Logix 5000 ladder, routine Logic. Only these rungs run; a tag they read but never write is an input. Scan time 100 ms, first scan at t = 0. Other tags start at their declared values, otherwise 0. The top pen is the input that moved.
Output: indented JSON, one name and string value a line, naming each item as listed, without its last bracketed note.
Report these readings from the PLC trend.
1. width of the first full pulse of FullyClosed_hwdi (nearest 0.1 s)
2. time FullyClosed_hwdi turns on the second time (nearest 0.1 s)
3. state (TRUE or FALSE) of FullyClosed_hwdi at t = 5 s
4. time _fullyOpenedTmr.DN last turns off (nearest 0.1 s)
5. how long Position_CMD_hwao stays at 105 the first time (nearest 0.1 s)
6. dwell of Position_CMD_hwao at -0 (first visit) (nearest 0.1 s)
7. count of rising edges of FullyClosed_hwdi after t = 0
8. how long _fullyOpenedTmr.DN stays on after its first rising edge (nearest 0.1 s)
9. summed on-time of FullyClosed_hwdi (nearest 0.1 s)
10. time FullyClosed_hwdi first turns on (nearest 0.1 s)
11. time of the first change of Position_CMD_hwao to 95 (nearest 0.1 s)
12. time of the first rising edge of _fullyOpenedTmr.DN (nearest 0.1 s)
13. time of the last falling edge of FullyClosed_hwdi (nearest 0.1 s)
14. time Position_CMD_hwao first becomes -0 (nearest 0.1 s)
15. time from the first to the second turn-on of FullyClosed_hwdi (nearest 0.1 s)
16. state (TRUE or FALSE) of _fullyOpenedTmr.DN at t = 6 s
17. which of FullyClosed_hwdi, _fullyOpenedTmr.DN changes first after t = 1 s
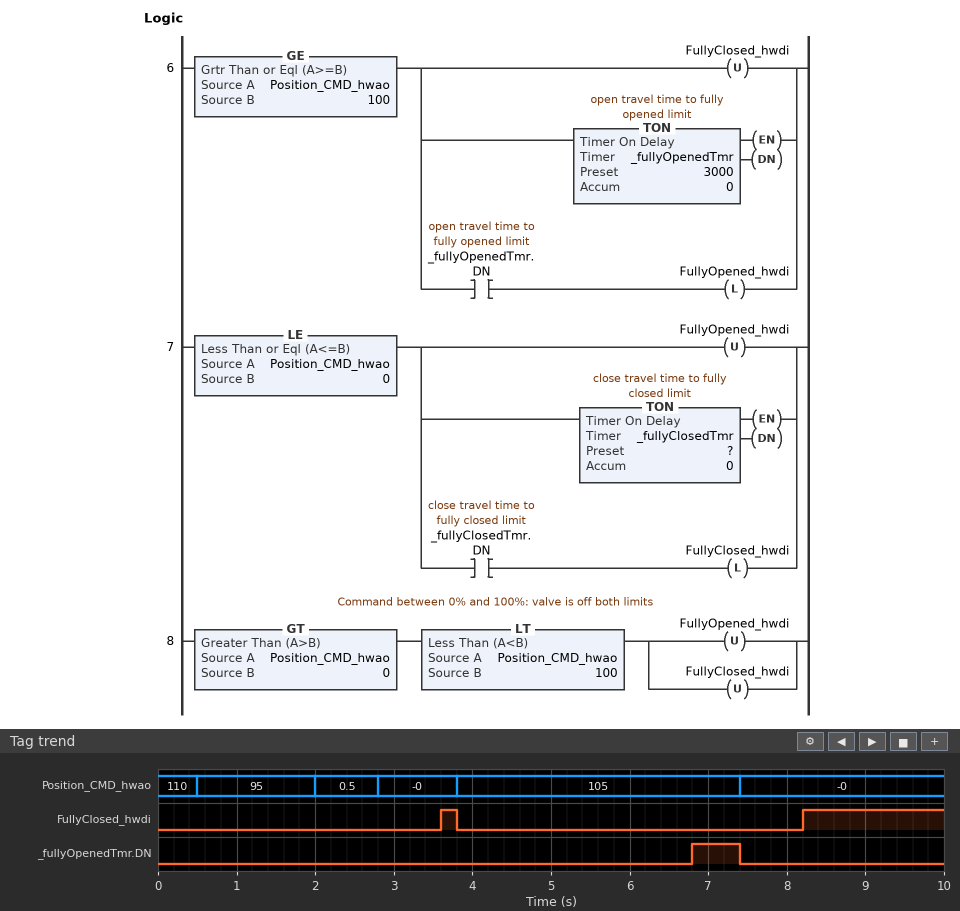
{
  "width of the first full pulse of FullyClosed_hwdi": "0.2 s",
  "time FullyClosed_hwdi turns on the second time": "8.2 s",
  "state (TRUE or FALSE) of FullyClosed_hwdi at t = 5 s": "FALSE",
  "time _fullyOpenedTmr.DN last turns off": "7.4 s",
  "how long Position_CMD_hwao stays at 105 the first time": "3.6 s",
  "dwell of Position_CMD_hwao at -0 (first visit)": "1.0 s",
  "count of rising edges of FullyClosed_hwdi after t = 0": "2",
  "how long _fullyOpenedTmr.DN stays on after its first rising edge": "0.6 s",
  "summed on-time of FullyClosed_hwdi": "2.0 s",
  "time FullyClosed_hwdi first turns on": "3.6 s",
  "time of the first change of Position_CMD_hwao to 95": "0.5 s",
  "time of the first rising edge of _fullyOpenedTmr.DN": "6.8 s",
  "time of the last falling edge of FullyClosed_hwdi": "3.8 s",
  "time Position_CMD_hwao first becomes -0": "2.8 s",
  "time from the first to the second turn-on of FullyClosed_hwdi": "4.6 s",
  "state (TRUE or FALSE) of _fullyOpenedTmr.DN at t = 6 s": "FALSE",
  "which of FullyClosed_hwdi, _fullyOpenedTmr.DN changes first after t = 1 s": "FullyClosed_hwdi"
}
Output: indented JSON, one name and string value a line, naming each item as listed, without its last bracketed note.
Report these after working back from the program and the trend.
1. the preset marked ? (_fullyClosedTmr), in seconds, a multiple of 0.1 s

{
  "the preset marked ? (_fullyClosedTmr), in seconds, a multiple of 0.1 s": "0.8 s"
}
